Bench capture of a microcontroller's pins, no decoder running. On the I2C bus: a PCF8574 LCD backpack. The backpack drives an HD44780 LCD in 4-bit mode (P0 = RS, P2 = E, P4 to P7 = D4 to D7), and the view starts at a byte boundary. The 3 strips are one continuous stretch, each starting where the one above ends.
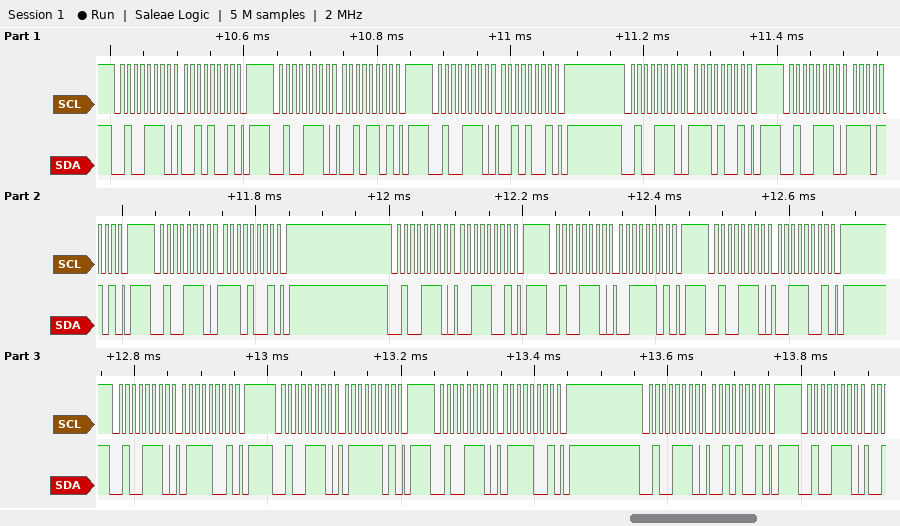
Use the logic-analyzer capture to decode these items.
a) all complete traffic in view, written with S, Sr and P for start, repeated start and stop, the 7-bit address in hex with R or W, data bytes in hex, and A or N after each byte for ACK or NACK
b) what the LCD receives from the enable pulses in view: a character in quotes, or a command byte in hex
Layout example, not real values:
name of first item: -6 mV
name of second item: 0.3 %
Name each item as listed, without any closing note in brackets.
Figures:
all complete traffic in view, written with S, Sr and P for start, repeated start and stop, the 7-bit address in hex with R or W, data bytes in hex, and A or N after each byte for ACK or NACK: S 27W A 29 A P S 27W A 2D A P S 27W A 29 A P S 27W A E9 A P S 27W A ED A P S 27W A E9 A P S 27W A 39 A P S 27W A 3D A P S 27W A 39 A P S 27W A 79 A P S 27W A 7D A P S 27W A 79 A P S 27W A 29 A P S 27W A
what the LCD receives from the enable pulses in view: a character in quotes, or a command byte in hex: '.' '7'
